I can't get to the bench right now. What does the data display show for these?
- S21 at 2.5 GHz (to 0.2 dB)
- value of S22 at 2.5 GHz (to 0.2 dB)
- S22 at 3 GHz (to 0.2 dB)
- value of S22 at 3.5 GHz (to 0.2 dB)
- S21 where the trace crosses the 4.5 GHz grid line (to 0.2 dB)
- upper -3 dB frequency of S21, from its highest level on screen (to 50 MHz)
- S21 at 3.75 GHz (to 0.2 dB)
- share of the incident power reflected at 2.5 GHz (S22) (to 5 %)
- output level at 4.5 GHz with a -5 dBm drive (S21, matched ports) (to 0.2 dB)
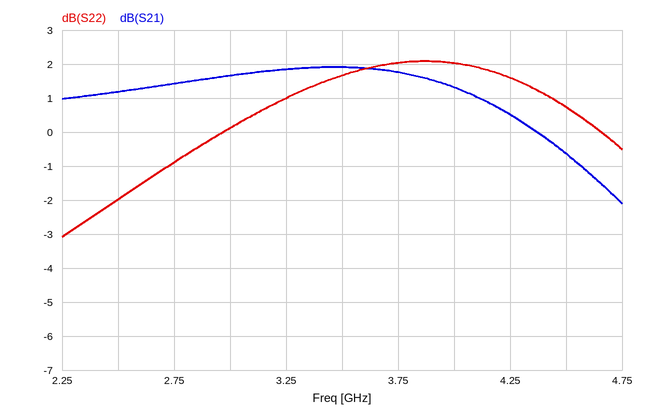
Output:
1.2 dB
-2.0 dB
0.2 dB
1.6 dB
-0.6 dB
4.60 GHz
1.8 dB
65 %
-5.6 dBm
